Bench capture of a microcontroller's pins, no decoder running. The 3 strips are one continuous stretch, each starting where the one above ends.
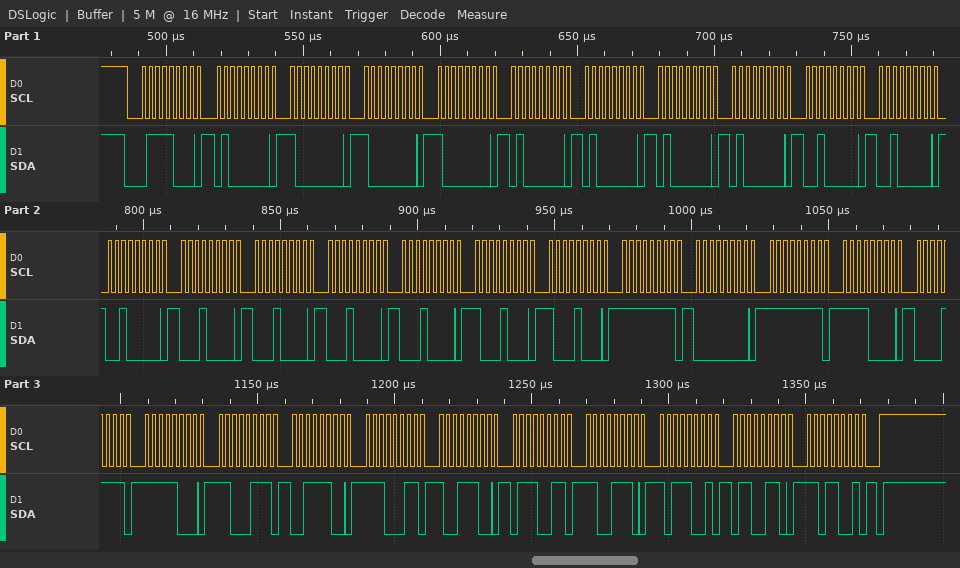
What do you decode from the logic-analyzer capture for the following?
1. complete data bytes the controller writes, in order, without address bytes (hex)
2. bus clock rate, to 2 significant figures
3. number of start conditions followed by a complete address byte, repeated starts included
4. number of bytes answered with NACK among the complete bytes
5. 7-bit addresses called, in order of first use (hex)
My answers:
40 80 80 80 40 40 40 40 20 20 20 10 10 10 10 88 88 FF 00 FF F0 0F F8 C7 3C E3 9C 73 CE B9 66 D9
400 kHz
1
0
0x3C
